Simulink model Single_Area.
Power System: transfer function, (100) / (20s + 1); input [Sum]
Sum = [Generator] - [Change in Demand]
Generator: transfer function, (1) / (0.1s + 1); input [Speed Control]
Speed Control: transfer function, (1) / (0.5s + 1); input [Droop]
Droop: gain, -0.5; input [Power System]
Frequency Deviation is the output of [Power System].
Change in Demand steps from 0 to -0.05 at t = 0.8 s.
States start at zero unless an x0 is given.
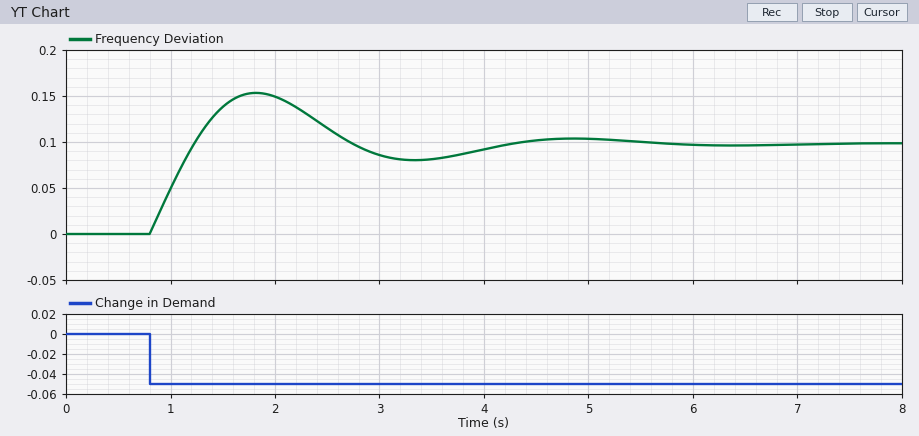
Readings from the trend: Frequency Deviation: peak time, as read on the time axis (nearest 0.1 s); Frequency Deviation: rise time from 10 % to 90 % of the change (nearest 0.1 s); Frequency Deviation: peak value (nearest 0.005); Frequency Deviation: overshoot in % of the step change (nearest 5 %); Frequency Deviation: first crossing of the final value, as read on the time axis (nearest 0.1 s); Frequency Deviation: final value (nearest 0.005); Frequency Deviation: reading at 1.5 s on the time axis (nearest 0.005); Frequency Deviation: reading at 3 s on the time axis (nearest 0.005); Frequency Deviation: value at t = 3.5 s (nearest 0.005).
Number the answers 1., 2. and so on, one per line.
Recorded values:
1. 1.8 s
2. 0.3 s
3. 0.155
4. 55 %
5. 1.2 s
6. 0.100
7. 0.140
8. 0.085
9. 0.080
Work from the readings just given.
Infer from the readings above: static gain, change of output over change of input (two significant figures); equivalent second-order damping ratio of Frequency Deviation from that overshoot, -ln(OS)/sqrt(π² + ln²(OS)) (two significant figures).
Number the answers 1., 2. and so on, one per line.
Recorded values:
1. -2.0
2. 0.19
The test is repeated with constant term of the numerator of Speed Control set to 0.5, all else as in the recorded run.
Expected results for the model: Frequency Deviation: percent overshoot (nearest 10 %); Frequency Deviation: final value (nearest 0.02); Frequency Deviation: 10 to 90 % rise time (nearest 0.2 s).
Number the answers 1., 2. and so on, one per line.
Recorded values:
1. 20 %
2. 0.20
3. 0.8 s
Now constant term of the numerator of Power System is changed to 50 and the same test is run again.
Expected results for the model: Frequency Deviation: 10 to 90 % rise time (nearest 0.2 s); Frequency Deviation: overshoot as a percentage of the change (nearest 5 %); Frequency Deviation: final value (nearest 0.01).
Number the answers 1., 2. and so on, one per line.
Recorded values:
1. 0.8 s
2. 20 %
3. 0.10
